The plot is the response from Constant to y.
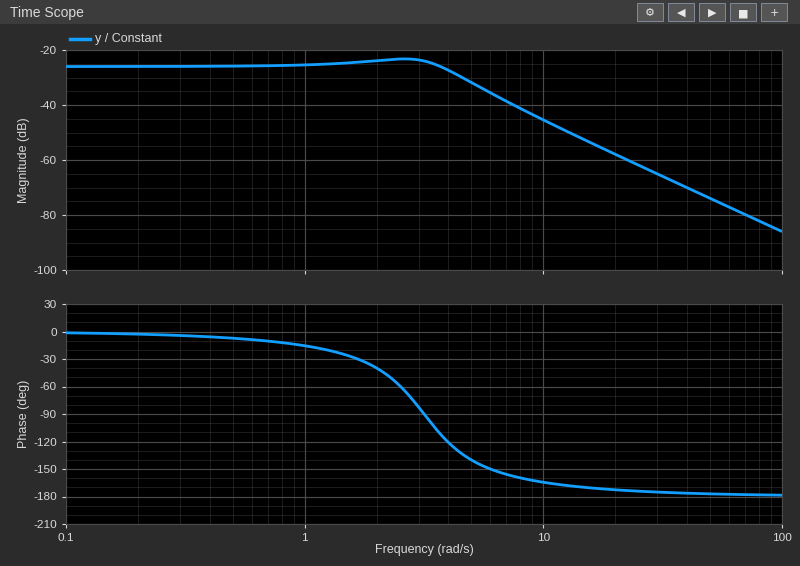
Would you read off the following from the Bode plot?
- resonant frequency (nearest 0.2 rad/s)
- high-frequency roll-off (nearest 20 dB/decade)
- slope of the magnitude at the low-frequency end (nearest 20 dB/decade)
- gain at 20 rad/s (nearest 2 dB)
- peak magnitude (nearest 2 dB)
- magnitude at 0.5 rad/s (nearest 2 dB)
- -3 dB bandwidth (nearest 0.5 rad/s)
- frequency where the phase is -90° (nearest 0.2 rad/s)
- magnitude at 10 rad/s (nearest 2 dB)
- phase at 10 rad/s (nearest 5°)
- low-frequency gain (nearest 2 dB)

2.6 rad/s
-40 dB/decade
0 dB/decade
-58 dB
-24 dB
-26 dB
4.5 rad/s
3.2 rad/s
-46 dB
-165°
-26 dB
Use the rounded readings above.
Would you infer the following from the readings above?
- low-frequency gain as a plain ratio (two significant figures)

0.050
